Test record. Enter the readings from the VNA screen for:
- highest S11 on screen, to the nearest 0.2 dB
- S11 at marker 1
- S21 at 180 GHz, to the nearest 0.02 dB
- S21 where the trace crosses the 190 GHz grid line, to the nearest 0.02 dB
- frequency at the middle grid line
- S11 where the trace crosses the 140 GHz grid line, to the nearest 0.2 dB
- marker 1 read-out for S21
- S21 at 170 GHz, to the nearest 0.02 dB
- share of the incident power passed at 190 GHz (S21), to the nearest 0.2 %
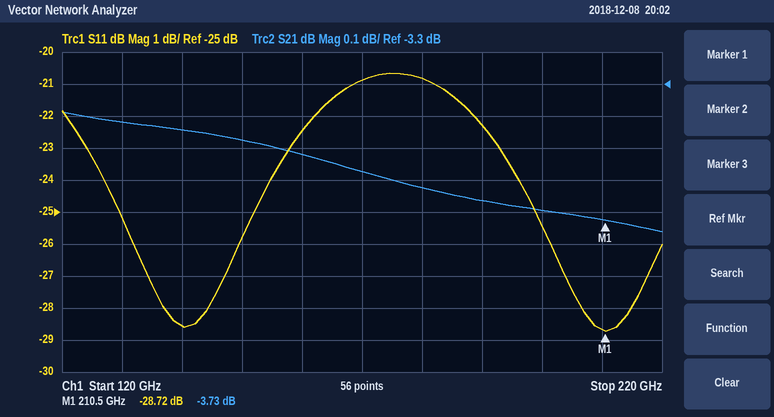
-20.6 dB
-28.72 dB
-3.62 dB
-3.66 dB
170 GHz
-28.6 dB
-3.73 dB
-3.58 dB
43.0 %
